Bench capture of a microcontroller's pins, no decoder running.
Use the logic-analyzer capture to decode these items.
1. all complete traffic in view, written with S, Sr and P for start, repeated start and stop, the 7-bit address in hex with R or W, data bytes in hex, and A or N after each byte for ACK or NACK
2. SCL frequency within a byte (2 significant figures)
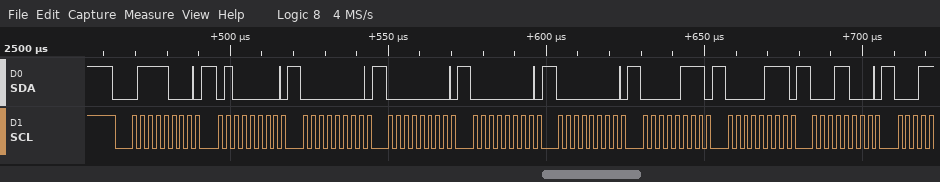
S 3CW A 40 A 00 A 00 A 00 A 00 A 07 A 07 A 18 A
400 kHz
